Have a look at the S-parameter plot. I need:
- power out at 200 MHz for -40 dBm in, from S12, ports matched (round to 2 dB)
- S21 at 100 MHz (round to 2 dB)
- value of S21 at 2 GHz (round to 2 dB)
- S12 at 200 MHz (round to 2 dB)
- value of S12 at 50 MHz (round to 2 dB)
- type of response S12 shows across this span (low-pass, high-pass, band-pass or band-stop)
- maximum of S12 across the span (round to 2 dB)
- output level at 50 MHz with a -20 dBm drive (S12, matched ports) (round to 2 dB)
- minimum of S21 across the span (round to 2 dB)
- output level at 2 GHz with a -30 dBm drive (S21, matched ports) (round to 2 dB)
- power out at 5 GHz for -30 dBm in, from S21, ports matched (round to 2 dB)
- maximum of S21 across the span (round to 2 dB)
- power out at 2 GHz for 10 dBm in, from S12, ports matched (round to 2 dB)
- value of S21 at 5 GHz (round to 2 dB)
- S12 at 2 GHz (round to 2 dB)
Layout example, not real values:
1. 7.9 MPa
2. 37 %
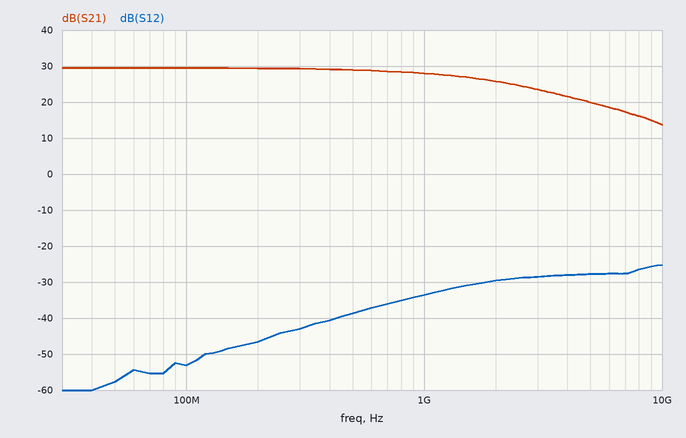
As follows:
1. -86 dBm
2. 30 dB
3. 26 dB
4. -46 dB
5. -58 dB
6. high-pass
7. -26 dB
8. -78 dBm
9. 14 dB
10. -4 dBm
11. -10 dBm
12. 30 dB
13. -20 dBm
14. 20 dB
15. -30 dB
